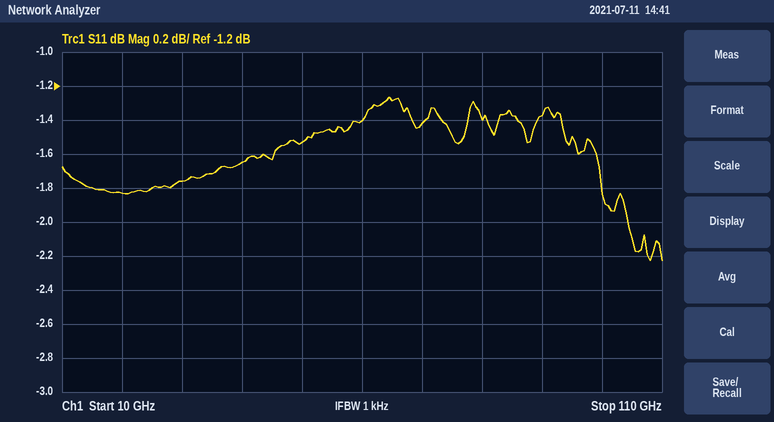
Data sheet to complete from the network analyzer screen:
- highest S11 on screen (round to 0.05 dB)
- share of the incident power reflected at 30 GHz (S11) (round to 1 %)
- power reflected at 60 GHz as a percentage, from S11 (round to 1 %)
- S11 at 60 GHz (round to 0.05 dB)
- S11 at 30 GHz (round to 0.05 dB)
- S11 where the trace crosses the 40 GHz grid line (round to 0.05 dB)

-1.25 dB
67 %
72 %
-1.40 dB
-1.75 dB
-1.65 dB
